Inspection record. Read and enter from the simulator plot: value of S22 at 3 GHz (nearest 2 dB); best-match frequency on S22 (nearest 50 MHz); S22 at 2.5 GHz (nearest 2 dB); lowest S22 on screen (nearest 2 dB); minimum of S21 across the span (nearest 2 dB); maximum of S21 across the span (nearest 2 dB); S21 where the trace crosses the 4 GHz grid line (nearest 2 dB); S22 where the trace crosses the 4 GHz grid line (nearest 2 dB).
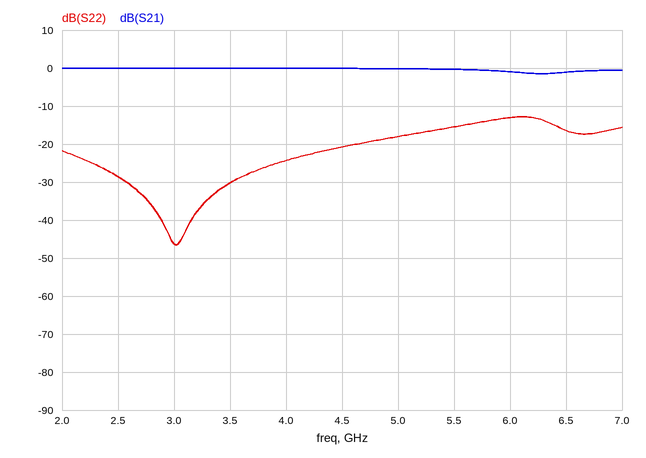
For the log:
-46 dB
3.00 GHz
-28 dB
-46 dB
-2 dB
0 dB
0 dB
-24 dB
